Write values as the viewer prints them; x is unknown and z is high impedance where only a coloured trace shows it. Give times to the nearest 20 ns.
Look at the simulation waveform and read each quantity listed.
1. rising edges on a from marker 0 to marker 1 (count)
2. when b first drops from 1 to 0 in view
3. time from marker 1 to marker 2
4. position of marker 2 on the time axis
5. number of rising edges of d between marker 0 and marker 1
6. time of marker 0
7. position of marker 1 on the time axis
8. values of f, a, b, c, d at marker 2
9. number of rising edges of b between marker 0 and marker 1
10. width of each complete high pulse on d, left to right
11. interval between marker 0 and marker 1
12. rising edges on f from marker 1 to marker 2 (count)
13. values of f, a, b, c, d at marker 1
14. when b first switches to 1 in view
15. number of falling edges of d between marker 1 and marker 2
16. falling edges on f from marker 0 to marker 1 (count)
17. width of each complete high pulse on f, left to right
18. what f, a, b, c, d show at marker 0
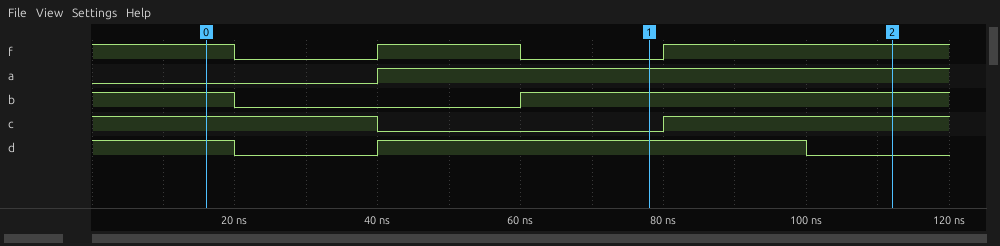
1
20 ns
40 ns
120 ns
1
20 ns
80 ns
f=1, a=1, b=1, c=1, d=0
1
60 ns
60 ns
1
f=0, a=1, b=1, c=0, d=1
60 ns
1
2
20 ns
f=1, a=0, b=1, c=1, d=1
